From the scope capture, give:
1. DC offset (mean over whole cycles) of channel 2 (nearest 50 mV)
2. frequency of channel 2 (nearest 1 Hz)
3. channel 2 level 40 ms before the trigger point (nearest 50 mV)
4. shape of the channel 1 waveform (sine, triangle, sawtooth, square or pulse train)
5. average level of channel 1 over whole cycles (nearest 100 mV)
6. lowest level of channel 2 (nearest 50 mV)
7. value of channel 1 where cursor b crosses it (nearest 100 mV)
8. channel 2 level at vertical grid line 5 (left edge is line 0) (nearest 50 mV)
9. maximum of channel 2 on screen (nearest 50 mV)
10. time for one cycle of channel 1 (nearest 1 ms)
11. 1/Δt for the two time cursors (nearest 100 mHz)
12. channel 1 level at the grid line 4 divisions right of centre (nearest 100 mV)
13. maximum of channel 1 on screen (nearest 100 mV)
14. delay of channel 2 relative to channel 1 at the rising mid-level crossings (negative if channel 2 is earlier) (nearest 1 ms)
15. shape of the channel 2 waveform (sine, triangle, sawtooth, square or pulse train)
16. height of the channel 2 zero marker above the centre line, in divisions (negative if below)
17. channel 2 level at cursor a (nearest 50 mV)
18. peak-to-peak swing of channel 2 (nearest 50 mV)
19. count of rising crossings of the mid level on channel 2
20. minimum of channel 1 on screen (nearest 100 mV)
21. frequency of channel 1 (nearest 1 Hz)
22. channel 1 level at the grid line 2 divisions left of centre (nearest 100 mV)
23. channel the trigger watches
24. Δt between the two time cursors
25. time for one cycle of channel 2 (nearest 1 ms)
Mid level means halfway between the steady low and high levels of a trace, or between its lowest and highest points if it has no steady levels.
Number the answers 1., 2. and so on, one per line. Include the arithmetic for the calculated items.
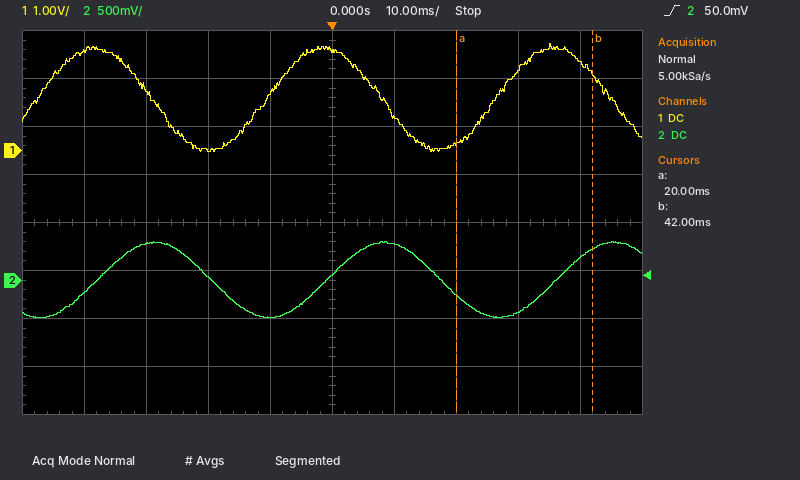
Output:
1. (400 mV + (-400 mV)) / 2 ≈ 0 mV
2. 1 / 37 ms ≈ 27 Hz
3. -150 mV
4. sine
5. (2.2 V + (0.0 V)) / 2 ≈ 1.1 V
6. -400 mV
7. 1.6 V
8. 50 mV
9. 400 mV
10. 37 ms
11. 1 / 22 ms ≈ 45.5 Hz
12. 1.8 V
13. 2.2 V
14. +10 ms
15. sine
16. -1.2 div
17. -150 mV
18. 400 mV − (-400 mV) = 800 mV
19. 3
20. 0.0 V
21. 1 / 37 ms ≈ 27 Hz
22. 0.0 V
23. channel 2
24. 42 ms − (20 ms) = 22 ms
25. 37 ms
